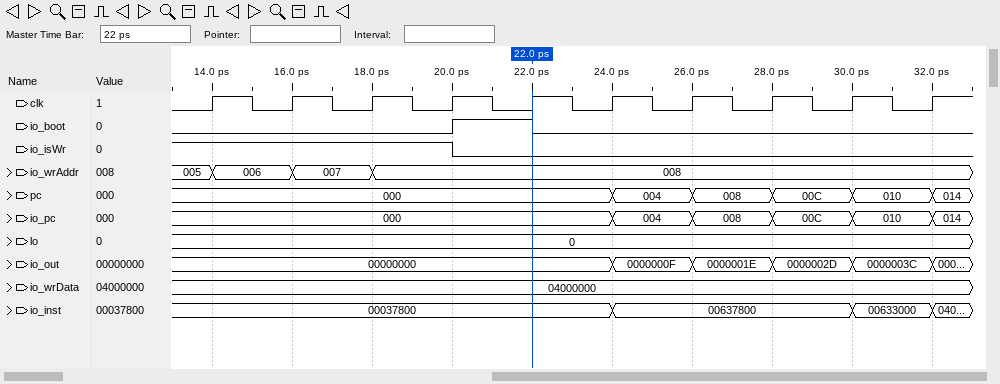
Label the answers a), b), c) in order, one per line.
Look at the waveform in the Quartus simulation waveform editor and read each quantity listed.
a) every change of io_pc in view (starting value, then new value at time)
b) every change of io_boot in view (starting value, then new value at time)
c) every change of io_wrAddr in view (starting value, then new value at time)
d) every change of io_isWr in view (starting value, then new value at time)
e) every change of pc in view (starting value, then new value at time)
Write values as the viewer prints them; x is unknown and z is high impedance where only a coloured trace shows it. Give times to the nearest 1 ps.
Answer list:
a) 000, 004 at 24 ps, 008 at 26 ps, 00C at 28 ps, 010 at 30 ps, 014 at 32 ps
b) 0, 1 at 20 ps, 0 at 22 ps
c) 005, 006 at 14 ps, 007 at 16 ps, 008 at 18 ps
d) 1, 0 at 20 ps
e) 000, 004 at 24 ps, 008 at 26 ps, 00C at 28 ps, 010 at 30 ps, 014 at 32 ps
